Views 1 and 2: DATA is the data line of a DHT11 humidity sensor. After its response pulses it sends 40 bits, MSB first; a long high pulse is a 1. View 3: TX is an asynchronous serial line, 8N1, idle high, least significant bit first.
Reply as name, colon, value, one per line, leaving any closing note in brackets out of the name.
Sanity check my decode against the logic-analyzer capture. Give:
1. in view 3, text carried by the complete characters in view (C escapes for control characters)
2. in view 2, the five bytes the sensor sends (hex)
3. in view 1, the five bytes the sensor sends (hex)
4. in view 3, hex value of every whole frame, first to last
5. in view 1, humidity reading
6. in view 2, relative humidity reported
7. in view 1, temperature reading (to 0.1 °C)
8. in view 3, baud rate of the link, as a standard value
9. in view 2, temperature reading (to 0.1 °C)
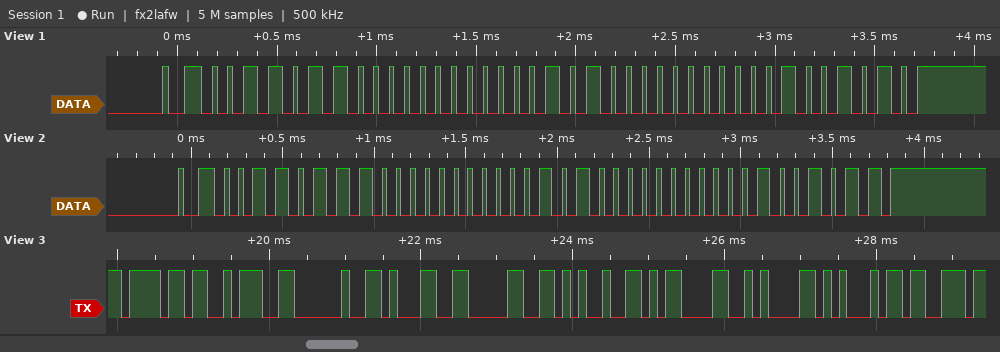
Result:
in view 3, text carried by the complete characters in view: "o: 10%\r\nEs"
in view 2, the five bytes the sensor sends: 37 00 14 00 4B
in view 1, the five bytes the sensor sends: 36 00 14 00 4A
in view 3, hex value of every whole frame, first to last: 6F 3A 20 31 30 25 0D 0A 45 73
in view 1, humidity reading: 54 %
in view 2, relative humidity reported: 55 %
in view 1, temperature reading: 20.0 °C
in view 3, baud rate of the link, as a standard value: 9600 baud
in view 2, temperature reading: 20.0 °C
